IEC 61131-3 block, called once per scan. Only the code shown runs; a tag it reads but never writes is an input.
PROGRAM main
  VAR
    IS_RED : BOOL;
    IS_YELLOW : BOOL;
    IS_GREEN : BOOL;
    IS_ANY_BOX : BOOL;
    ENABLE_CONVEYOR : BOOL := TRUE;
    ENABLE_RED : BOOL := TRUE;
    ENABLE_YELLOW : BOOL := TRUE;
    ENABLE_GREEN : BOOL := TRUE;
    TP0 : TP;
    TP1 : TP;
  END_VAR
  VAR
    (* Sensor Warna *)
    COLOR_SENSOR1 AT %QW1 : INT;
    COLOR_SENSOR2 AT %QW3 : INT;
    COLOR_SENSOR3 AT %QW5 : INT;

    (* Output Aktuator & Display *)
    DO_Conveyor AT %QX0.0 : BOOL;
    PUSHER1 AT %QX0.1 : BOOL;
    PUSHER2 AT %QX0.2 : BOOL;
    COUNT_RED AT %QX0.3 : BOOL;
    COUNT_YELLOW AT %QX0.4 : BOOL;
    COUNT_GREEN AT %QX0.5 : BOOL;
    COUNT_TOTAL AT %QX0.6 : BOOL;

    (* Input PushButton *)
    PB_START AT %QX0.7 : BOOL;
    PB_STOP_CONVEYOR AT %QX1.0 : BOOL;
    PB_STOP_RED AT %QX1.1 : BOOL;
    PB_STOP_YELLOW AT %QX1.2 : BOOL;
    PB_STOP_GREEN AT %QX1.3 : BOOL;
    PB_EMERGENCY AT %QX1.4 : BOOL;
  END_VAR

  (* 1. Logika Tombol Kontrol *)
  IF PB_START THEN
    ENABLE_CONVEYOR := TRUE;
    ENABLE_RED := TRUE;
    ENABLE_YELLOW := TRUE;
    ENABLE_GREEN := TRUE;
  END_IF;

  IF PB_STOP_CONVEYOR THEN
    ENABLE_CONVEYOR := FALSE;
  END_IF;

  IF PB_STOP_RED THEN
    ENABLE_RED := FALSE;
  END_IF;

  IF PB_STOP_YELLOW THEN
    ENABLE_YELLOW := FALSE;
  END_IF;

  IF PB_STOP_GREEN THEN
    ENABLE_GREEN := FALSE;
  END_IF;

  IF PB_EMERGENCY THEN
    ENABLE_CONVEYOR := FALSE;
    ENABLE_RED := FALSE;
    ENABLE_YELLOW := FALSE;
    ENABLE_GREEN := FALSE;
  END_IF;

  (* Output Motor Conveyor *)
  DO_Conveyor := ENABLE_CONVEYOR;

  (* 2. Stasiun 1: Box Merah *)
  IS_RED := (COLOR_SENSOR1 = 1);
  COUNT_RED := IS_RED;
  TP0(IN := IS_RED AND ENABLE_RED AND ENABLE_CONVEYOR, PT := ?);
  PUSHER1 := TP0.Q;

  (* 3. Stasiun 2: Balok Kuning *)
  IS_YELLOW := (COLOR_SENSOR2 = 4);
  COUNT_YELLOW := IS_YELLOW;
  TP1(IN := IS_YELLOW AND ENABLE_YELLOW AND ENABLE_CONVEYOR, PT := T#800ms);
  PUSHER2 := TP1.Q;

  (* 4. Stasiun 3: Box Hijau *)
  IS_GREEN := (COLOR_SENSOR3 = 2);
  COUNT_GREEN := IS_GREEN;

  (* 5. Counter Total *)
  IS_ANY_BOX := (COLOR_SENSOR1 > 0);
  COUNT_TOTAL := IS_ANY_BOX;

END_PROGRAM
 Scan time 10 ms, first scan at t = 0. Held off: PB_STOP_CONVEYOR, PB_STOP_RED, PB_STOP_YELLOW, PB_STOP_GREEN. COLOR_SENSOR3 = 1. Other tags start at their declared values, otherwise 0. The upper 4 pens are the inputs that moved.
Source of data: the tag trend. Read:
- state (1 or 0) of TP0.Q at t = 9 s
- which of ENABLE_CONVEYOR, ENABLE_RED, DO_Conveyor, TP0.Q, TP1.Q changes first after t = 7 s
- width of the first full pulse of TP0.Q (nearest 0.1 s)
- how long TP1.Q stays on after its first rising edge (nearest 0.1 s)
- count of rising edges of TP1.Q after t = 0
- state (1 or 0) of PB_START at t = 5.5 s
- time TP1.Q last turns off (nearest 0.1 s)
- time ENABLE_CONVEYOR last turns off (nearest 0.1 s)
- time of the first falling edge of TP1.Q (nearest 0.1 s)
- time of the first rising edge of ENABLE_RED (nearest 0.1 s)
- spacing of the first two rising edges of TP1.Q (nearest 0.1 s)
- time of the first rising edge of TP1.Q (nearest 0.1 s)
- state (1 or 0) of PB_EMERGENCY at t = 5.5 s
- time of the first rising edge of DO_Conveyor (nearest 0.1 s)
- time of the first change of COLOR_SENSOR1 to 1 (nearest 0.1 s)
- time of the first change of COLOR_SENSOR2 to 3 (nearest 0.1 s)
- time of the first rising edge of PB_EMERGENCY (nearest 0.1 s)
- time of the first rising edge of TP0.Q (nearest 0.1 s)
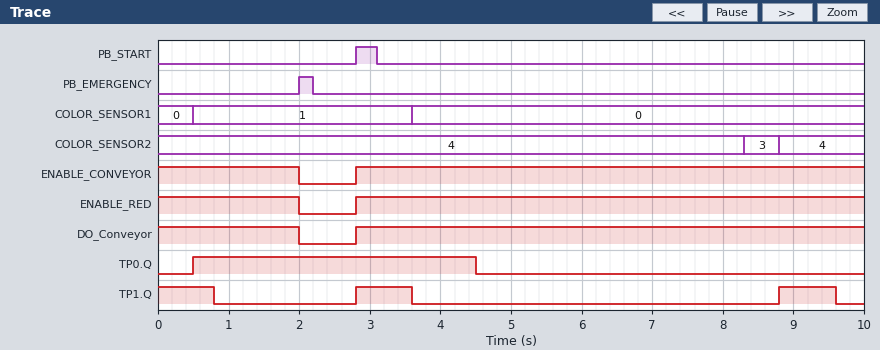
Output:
0
TP1.Q
4.0 s
0.8 s
2
0
9.6 s
2.0 s
0.8 s
2.8 s
6.0 s
2.8 s
0
2.8 s
0.5 s
8.3 s
2.0 s
0.5 s
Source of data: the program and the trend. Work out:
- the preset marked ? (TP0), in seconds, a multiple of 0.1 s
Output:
4.0 s
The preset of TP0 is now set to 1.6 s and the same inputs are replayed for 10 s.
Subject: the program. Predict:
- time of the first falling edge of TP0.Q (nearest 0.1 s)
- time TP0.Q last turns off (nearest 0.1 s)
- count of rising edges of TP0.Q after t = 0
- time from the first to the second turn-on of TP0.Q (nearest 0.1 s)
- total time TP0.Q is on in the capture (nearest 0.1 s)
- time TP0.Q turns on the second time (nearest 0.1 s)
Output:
2.1 s
4.4 s
2
2.3 s
3.2 s
2.8 s
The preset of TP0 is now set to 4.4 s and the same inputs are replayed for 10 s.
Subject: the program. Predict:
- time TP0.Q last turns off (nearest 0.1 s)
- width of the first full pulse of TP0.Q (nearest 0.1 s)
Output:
4.9 s
4.4 s
